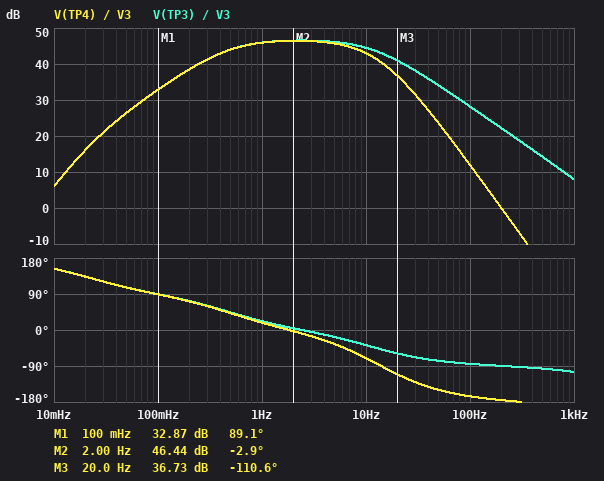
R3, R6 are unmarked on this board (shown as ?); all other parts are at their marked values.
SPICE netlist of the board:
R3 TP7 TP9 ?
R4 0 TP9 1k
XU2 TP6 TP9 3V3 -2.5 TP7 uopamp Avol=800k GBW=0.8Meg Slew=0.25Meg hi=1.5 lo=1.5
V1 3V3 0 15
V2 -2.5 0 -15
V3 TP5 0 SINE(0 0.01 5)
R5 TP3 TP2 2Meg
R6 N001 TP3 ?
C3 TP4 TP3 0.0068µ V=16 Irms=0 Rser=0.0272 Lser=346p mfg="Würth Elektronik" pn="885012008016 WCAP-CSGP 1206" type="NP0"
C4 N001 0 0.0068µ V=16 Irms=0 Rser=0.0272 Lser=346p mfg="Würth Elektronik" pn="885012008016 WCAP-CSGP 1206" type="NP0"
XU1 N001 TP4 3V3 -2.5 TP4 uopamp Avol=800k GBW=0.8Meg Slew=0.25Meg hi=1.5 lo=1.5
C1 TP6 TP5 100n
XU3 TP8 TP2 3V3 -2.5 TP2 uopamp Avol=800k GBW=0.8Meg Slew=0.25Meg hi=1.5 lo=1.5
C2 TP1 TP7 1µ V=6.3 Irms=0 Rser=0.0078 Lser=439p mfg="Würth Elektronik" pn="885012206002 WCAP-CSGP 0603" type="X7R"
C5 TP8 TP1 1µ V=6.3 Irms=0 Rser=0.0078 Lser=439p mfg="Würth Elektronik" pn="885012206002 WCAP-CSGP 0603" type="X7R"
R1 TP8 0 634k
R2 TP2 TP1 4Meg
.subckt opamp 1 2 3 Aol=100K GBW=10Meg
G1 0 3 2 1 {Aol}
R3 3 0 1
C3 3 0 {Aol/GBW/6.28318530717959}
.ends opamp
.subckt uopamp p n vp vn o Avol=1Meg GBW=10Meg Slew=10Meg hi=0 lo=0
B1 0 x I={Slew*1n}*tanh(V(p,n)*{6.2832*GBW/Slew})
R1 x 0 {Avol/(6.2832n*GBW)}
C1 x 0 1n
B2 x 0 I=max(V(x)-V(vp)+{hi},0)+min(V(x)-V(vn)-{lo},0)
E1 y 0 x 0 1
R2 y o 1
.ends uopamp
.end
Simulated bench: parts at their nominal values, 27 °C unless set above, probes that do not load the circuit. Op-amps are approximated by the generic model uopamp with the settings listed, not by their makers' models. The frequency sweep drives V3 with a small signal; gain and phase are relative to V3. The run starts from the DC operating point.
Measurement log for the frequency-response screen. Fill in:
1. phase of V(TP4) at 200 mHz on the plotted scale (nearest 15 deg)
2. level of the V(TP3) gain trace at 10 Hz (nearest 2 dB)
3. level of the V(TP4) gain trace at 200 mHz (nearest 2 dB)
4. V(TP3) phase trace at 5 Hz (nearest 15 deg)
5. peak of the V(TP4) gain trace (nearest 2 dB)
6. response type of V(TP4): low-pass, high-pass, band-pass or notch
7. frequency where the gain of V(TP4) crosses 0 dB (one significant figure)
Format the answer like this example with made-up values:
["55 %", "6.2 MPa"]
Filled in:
["75 deg", "44 dB", "38 dB", "-15 deg", "46 dB", "band-pass", "200 Hz"]
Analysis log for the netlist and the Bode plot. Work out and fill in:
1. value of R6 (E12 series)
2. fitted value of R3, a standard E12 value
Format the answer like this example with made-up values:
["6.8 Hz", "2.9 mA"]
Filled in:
["1.5 MΩ", "220 kΩ"]
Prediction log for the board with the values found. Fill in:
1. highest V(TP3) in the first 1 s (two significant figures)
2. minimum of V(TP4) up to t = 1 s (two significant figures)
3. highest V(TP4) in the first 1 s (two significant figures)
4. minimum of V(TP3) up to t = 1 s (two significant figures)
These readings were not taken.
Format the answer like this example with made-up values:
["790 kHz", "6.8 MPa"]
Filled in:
["2.0 V", "-2.1 V", "1.9 V", "-2.2 V"]
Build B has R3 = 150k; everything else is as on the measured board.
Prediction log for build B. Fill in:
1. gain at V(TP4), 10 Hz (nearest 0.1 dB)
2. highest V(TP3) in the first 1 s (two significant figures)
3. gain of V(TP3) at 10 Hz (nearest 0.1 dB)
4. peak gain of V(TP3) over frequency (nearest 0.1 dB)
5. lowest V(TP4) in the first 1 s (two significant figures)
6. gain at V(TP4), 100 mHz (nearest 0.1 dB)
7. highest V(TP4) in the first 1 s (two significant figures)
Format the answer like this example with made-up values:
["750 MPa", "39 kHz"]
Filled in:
["39.7 dB", "1.4 V", "41.2 dB", "43.2 dB", "-1.4 V", "29.6 dB", "1.3 V"]
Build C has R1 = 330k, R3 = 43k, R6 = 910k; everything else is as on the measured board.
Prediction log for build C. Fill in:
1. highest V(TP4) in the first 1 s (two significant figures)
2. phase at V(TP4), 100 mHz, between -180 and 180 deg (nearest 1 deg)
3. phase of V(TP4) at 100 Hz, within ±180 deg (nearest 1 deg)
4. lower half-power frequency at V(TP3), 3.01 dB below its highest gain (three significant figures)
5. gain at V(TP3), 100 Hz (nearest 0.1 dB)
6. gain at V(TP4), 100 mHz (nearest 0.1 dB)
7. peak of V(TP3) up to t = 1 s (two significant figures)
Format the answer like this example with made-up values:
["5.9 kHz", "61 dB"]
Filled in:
["390 mV", "95 deg", "-159 deg", "821 mHz", "14.2 dB", "13.1 dB", "400 mV"]
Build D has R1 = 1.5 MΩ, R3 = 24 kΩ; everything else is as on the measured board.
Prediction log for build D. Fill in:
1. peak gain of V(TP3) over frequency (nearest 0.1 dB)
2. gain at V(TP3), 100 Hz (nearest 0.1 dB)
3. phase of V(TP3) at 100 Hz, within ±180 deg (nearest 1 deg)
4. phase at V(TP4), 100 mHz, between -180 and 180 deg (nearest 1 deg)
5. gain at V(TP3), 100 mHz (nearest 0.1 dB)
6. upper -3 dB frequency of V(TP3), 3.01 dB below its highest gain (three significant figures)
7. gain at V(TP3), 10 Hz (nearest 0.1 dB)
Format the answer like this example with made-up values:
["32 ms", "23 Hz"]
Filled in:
["27.8 dB", "9.3 dB", "-83 deg", "74 deg", "21.1 dB", "12.1 Hz", "25.6 dB"]
